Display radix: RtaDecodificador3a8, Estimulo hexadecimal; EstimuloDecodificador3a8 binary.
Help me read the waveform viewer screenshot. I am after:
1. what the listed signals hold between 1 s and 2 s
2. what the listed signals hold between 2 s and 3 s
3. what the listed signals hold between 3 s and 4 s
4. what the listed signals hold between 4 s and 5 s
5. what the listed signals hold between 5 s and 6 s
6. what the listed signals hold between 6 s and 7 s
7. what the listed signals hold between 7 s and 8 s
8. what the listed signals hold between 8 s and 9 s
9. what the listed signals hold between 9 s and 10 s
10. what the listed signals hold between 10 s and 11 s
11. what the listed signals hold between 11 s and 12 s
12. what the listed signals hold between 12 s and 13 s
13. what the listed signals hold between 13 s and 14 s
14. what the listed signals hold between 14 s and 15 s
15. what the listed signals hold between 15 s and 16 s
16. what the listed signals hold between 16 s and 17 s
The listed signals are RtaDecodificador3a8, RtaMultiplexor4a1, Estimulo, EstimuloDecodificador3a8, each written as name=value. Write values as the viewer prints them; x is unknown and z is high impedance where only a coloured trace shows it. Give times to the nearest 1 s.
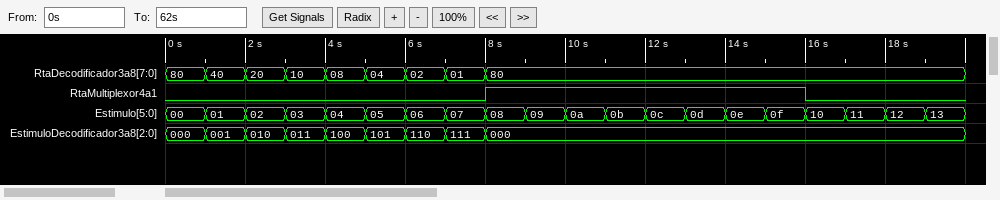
RtaDecodificador3a8=40, RtaMultiplexor4a1=0, Estimulo=01, EstimuloDecodificador3a8=001
RtaDecodificador3a8=20, RtaMultiplexor4a1=0, Estimulo=02, EstimuloDecodificador3a8=010
RtaDecodificador3a8=10, RtaMultiplexor4a1=0, Estimulo=03, EstimuloDecodificador3a8=011
RtaDecodificador3a8=08, RtaMultiplexor4a1=0, Estimulo=04, EstimuloDecodificador3a8=100
RtaDecodificador3a8=04, RtaMultiplexor4a1=0, Estimulo=05, EstimuloDecodificador3a8=101
RtaDecodificador3a8=02, RtaMultiplexor4a1=0, Estimulo=06, EstimuloDecodificador3a8=110
RtaDecodificador3a8=01, RtaMultiplexor4a1=0, Estimulo=07, EstimuloDecodificador3a8=111
RtaDecodificador3a8=80, RtaMultiplexor4a1=1, Estimulo=08, EstimuloDecodificador3a8=000
RtaDecodificador3a8=80, RtaMultiplexor4a1=1, Estimulo=09, EstimuloDecodificador3a8=000
RtaDecodificador3a8=80, RtaMultiplexor4a1=1, Estimulo=0a, EstimuloDecodificador3a8=000
RtaDecodificador3a8=80, RtaMultiplexor4a1=1, Estimulo=0b, EstimuloDecodificador3a8=000
RtaDecodificador3a8=80, RtaMultiplexor4a1=1, Estimulo=0c, EstimuloDecodificador3a8=000
RtaDecodificador3a8=80, RtaMultiplexor4a1=1, Estimulo=0d, EstimuloDecodificador3a8=000
RtaDecodificador3a8=80, RtaMultiplexor4a1=1, Estimulo=0e, EstimuloDecodificador3a8=000
RtaDecodificador3a8=80, RtaMultiplexor4a1=1, Estimulo=0f, EstimuloDecodificador3a8=000
RtaDecodificador3a8=80, RtaMultiplexor4a1=0, Estimulo=10, EstimuloDecodificador3a8=000
